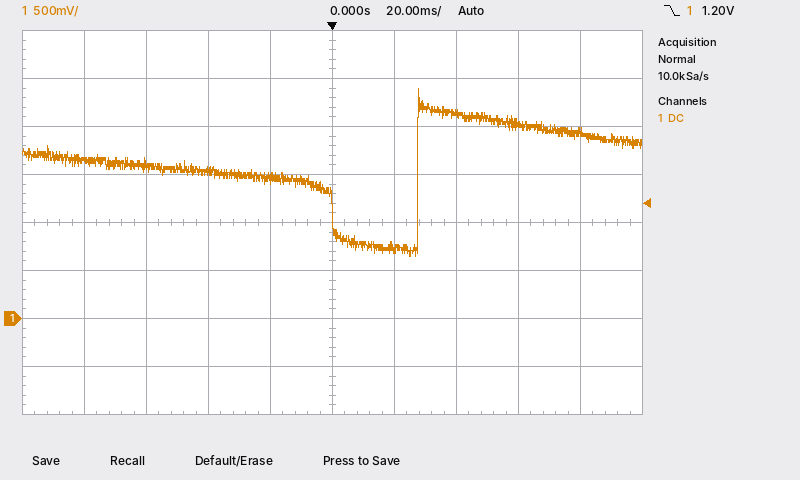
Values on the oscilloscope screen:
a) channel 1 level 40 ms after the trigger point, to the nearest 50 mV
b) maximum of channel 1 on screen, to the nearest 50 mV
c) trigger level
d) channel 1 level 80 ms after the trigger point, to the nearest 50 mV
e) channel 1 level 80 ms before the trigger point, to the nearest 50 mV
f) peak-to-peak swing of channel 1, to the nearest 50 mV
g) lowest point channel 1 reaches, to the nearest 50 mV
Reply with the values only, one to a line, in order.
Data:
2.15 V
2.40 V
1.20 V
1.95 V
1.65 V
1.75 V
650 mV
